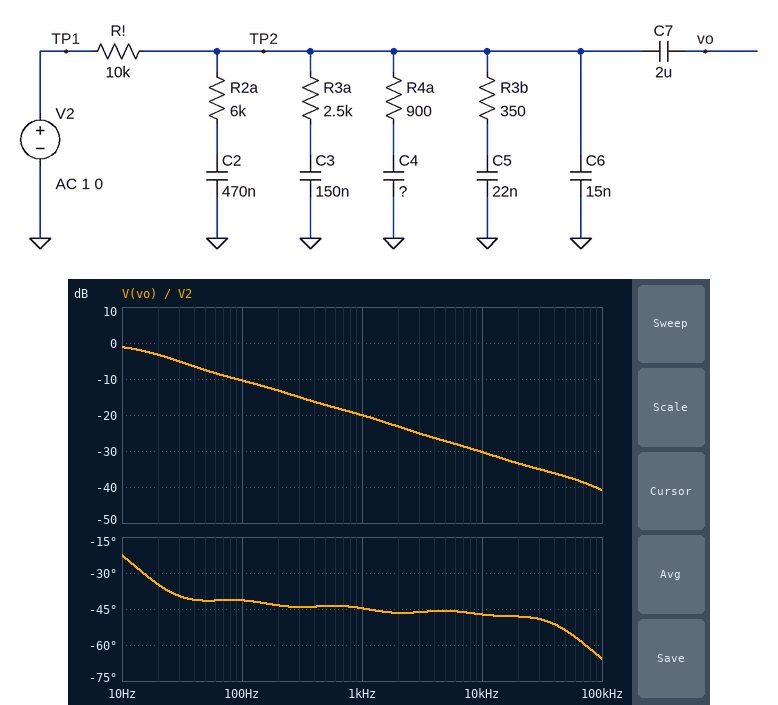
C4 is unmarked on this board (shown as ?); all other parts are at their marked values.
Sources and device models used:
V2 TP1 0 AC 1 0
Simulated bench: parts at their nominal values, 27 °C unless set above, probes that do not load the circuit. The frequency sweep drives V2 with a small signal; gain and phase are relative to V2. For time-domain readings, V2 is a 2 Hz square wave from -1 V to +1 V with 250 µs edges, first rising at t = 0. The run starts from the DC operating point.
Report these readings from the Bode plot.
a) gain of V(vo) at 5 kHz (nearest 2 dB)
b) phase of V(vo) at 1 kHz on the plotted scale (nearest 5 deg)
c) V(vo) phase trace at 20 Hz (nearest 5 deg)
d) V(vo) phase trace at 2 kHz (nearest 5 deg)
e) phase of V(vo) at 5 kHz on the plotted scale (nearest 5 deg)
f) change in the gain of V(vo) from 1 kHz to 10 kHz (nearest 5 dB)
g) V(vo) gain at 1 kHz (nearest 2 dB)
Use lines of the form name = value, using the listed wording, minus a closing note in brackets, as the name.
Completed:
gain of V(vo) at 5 kHz = -28 dB
phase of V(vo) at 1 kHz on the plotted scale = -45 deg
V(vo) phase trace at 20 Hz = -35 deg
V(vo) phase trace at 2 kHz = -45 deg
phase of V(vo) at 5 kHz on the plotted scale = -45 deg
change in the gain of V(vo) from 1 kHz to 10 kHz = -10 dB
V(vo) gain at 1 kHz = -20 dB
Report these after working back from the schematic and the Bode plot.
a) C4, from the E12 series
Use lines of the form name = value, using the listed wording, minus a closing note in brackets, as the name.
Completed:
C4, from the E12 series = 56 nF
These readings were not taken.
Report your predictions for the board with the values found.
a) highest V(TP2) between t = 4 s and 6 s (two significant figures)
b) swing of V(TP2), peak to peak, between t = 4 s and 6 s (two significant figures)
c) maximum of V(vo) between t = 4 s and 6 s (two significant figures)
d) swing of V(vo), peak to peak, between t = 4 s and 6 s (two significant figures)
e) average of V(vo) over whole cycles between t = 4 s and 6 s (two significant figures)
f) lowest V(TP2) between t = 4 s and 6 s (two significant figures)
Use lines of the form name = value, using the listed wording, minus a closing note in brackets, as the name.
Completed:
highest V(TP2) between t = 4 s and 6 s = 1.0 V
swing of V(TP2), peak to peak, between t = 4 s and 6 s = 2.0 V
maximum of V(vo) between t = 4 s and 6 s = 2.0 V
swing of V(vo), peak to peak, between t = 4 s and 6 s = 2.0 V
average of V(vo) over whole cycles between t = 4 s and 6 s = 1.0 V
lowest V(TP2) between t = 4 s and 6 s = -1.0 V
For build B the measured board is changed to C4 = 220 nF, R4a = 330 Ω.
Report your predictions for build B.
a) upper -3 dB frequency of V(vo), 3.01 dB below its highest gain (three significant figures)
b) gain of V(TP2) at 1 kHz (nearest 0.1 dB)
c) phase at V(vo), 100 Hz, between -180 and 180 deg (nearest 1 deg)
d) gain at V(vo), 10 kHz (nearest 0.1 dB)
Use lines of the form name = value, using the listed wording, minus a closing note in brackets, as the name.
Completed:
upper -3 dB frequency of V(vo), 3.01 dB below its highest gain = 16.0 Hz
gain of V(TP2) at 1 kHz = -25.6 dB
phase at V(vo), 100 Hz, between -180 and 180 deg = -52 deg
gain at V(vo), 10 kHz = -33.8 dB
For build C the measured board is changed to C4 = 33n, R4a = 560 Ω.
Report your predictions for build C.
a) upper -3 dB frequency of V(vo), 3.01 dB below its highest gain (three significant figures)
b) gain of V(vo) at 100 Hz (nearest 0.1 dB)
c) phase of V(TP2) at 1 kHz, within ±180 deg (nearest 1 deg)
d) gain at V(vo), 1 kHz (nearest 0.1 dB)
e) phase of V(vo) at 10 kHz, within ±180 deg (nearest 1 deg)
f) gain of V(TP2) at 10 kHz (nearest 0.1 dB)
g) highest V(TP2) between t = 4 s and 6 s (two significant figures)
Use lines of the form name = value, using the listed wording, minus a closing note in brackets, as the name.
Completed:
upper -3 dB frequency of V(vo), 3.01 dB below its highest gain = 19.3 Hz
gain of V(vo) at 100 Hz = -10.1 dB
phase of V(TP2) at 1 kHz, within ±180 deg = -43 deg
gain at V(vo), 1 kHz = -18.8 dB
phase of V(vo) at 10 kHz, within ±180 deg = -53 deg
gain of V(TP2) at 10 kHz = -31.4 dB
highest V(TP2) between t = 4 s and 6 s = 1.0 V
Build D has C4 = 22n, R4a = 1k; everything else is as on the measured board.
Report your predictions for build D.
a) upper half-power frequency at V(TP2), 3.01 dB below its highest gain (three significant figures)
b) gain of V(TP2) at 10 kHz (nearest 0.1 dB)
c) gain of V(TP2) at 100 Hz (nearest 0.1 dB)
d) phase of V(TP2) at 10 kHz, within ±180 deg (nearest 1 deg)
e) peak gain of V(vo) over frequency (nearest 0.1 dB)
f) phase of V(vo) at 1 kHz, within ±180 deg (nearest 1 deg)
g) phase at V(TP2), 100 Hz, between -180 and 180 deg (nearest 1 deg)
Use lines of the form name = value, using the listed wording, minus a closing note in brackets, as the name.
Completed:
upper half-power frequency at V(TP2), 3.01 dB below its highest gain = 19.5 Hz
gain of V(TP2) at 10 kHz = -30.0 dB
gain of V(TP2) at 100 Hz = -10.0 dB
phase of V(TP2) at 10 kHz, within ±180 deg = -54 deg
peak gain of V(vo) over frequency = 0 dB
phase of V(vo) at 1 kHz, within ±180 deg = -40 deg
phase at V(TP2), 100 Hz, between -180 and 180 deg = -39 deg
